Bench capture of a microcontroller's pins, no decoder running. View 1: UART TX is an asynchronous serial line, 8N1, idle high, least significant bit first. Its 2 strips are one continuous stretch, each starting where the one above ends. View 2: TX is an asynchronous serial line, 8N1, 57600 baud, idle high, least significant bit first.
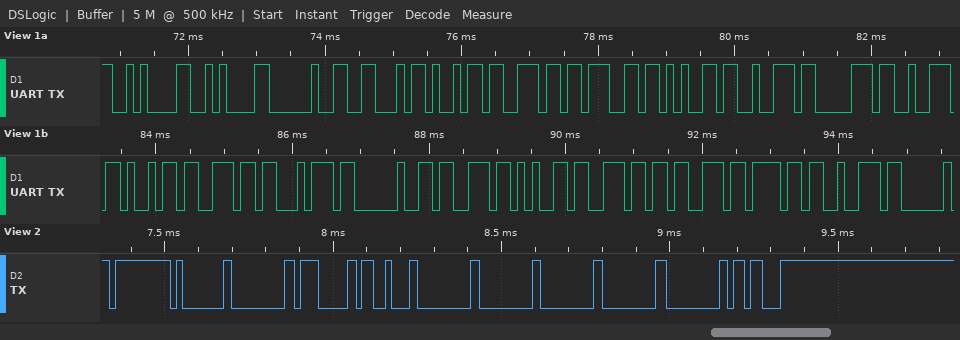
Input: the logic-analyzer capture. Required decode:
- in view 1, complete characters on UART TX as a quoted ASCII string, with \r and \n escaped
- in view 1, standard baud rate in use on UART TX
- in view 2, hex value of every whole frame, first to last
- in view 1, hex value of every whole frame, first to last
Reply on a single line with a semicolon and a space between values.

"\n\n Fingerprint sensor"; 9600 baud; FF 01 00 07 13 00 00 00 00 00 1B; 0x0A 0x0A 0x20 0x46 0x69 0x6E 0x67 0x65 0x72 0x70 0x72 0x69 0x6E 0x74 0x20 0x73 0x65 0x6E 0x73 0x6F 0x72
